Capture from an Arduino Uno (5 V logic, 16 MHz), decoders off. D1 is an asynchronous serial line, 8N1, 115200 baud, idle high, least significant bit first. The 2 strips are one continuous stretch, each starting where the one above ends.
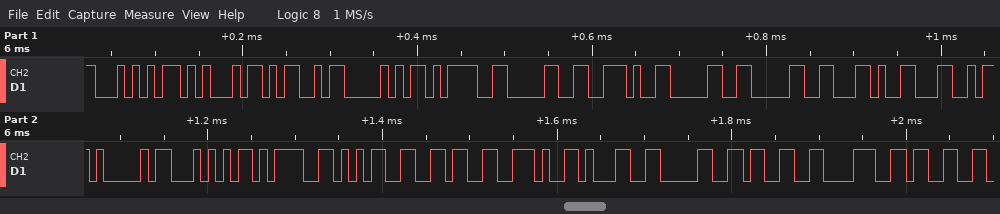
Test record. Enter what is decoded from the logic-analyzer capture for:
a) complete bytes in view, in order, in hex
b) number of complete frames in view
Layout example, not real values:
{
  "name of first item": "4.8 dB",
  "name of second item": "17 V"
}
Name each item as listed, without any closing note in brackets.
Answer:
{
  "complete bytes in view, in order, in hex": "54 45 4D 50 3D 30 2E 30 30 2C 4C 41 54 3D 35 36 2E 31 30 33 38 33",
  "number of complete frames in view": "22"
}
